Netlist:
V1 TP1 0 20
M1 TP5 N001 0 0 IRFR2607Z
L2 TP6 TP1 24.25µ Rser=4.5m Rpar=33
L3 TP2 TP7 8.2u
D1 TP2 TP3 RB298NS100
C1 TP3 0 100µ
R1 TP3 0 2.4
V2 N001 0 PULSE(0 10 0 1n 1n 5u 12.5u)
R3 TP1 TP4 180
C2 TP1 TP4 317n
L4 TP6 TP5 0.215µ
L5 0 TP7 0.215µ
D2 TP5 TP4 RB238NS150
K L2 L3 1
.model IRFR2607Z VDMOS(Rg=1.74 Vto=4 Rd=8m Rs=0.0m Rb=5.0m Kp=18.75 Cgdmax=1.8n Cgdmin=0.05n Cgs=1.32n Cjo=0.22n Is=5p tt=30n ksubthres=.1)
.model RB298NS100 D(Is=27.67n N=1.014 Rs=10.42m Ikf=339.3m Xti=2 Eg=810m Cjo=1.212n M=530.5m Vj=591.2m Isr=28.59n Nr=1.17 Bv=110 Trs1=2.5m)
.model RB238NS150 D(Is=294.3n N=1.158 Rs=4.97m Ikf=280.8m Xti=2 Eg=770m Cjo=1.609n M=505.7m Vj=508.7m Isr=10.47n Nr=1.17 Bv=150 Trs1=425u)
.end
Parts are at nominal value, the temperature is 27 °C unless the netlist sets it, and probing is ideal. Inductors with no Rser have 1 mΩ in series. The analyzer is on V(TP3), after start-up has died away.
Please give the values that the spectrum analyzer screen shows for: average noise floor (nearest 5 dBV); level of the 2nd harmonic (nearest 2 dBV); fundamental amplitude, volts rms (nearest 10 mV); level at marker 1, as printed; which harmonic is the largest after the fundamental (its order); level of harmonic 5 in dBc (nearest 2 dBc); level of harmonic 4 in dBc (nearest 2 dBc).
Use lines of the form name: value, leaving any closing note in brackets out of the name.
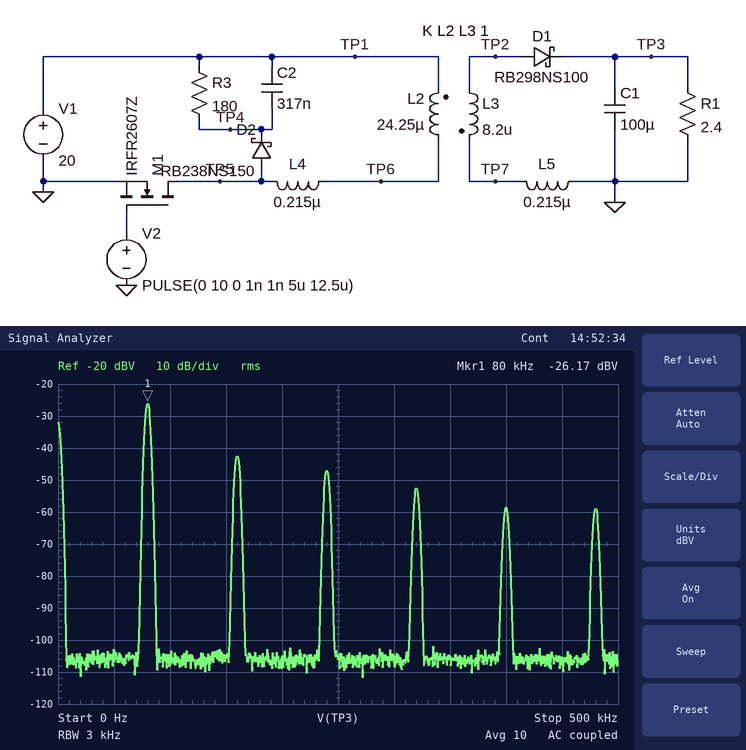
average noise floor: -105 dBV
level of the 2nd harmonic: -42 dBV
fundamental amplitude, volts rms: 50 mV
level at marker 1, as printed: -26.17 dBV
which harmonic is the largest after the fundamental: 2
level of harmonic 5 in dBc: -32 dBc
level of harmonic 4 in dBc: -26 dBc
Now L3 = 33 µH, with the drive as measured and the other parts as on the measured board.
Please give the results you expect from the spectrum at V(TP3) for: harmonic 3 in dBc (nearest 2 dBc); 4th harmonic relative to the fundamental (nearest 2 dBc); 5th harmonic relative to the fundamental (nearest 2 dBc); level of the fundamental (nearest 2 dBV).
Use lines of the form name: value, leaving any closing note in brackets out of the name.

harmonic 3 in dBc: -22 dBc
4th harmonic relative to the fundamental: -24 dBc
5th harmonic relative to the fundamental: -42 dBc
level of the fundamental: -22 dBV
